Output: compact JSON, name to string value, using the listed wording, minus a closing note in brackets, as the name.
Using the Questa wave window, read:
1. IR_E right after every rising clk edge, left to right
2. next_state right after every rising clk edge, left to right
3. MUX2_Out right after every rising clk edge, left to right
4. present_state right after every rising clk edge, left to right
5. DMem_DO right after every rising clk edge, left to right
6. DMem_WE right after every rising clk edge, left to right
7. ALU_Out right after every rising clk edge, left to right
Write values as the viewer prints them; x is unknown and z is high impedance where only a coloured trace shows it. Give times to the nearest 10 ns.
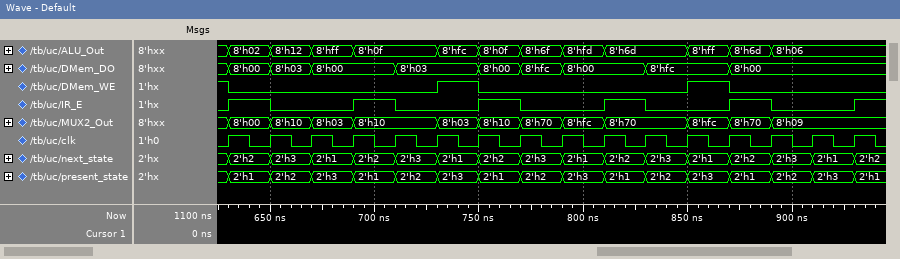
{"IR_E right after every rising clk edge, left to right": "1 0 0 1 0 0 1 0 0 1 0 0 1 0 0 1", "next_state right after every rising clk edge, left to right": "2'h2, 2'h3, 2'h1, 2'h2, 2'h3, 2'h1, 2'h2, 2'h3, 2'h1, 2'h2, 2'h3, 2'h1, 2'h2, 2'h3, 2'h1, 2'h2", "MUX2_Out right after every rising clk edge, left to right": "8'h00, 8'h10, 8'h03, 8'h10, 8'h10, 8'h03, 8'h10, 8'h70, 8'hfc, 8'h70, 8'h70, 8'hfc, 8'h70, 8'h09, 8'h09, 8'h09", "present_state right after every rising clk edge, left to right": "2'h1, 2'h2, 2'h3, 2'h1, 2'h2, 2'h3, 2'h1, 2'h2, 2'h3, 2'h1, 2'h2, 2'h3, 2'h1, 2'h2, 2'h3, 2'h1", "DMem_DO right after every rising clk edge, left to right": "8'h00, 8'h03, 8'h00, 8'h00, 8'h03, 8'h03, 8'h00, 8'hfc, 8'h00, 8'h00, 8'hfc, 8'hfc, 8'h00, 8'h00, 8'h00, 8'h00", "DMem_WE right after every rising clk edge, left to right": "0 0 0 0 0 1 0 0 0 0 0 1 0 0 0 0", "ALU_Out right after every rising clk edge, left to right": "8'h02, 8'h12, 8'hff, 8'h0f, 8'h0f, 8'hfc, 8'h0f, 8'h6f, 8'hfd, 8'h6d, 8'h6d, 8'hff, 8'h6d, 8'h06, 8'h06, 8'h06"}
